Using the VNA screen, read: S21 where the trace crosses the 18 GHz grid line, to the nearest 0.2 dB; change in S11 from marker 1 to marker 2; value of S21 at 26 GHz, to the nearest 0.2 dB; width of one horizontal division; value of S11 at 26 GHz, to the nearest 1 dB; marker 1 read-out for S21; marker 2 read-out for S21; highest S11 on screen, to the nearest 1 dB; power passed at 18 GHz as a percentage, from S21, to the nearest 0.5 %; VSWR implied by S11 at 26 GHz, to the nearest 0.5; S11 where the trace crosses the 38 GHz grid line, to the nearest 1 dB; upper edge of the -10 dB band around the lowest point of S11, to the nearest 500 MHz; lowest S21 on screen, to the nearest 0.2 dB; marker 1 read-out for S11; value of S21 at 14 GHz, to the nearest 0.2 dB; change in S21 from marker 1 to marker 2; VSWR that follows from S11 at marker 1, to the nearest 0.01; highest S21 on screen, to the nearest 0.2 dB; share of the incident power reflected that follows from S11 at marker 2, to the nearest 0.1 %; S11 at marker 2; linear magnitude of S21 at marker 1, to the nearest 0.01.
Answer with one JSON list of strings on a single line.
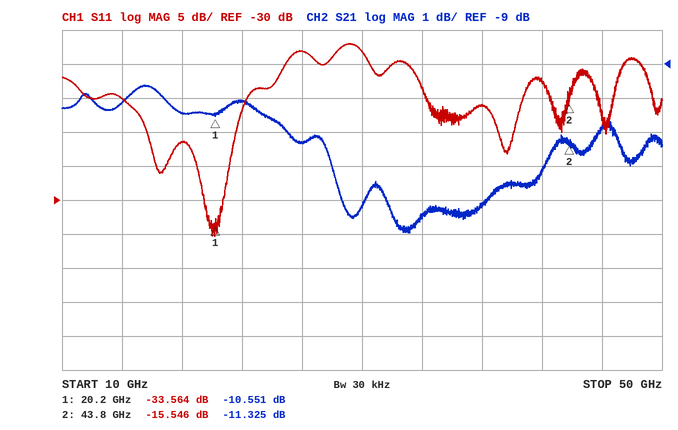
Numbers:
["-10.4 dB", "18.018 dB", "-11.4 dB", "4 GHz", "-8 dB", "-10.551 dB", "-11.325 dB", "-7 dB", "9.0 %", "2.5", "-16 dB", "25.0 GHz", "-14.0 dB", "-33.564 dB", "-10.2 dB", "-0.774 dB", "1.04", "-9.6 dB", "2.8 %", "-15.546 dB", "0.30"]
